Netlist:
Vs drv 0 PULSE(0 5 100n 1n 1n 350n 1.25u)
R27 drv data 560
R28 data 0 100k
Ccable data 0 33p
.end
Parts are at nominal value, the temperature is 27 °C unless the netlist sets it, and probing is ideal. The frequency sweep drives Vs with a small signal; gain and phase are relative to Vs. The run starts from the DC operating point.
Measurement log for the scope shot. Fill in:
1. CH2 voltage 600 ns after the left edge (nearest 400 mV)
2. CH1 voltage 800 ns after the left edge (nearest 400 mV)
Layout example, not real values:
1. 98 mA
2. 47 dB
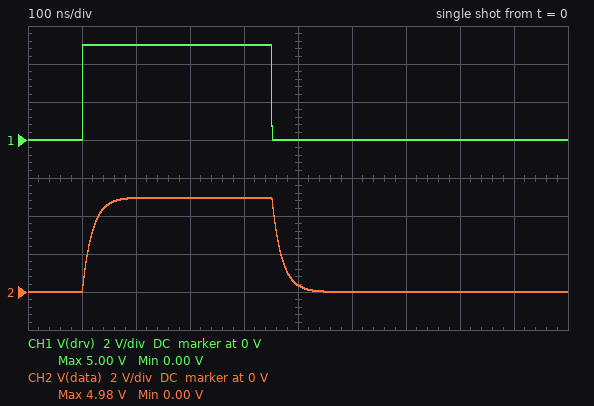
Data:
1. 0 V
2. 0 V
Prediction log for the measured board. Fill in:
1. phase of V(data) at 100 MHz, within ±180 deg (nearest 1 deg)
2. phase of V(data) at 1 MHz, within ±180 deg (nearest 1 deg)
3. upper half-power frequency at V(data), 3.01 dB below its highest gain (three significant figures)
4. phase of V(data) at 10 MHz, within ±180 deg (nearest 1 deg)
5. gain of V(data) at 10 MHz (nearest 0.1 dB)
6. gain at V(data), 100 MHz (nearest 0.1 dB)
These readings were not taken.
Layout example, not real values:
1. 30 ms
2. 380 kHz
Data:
1. -85 deg
2. -7 deg
3. 8.66 MHz
4. -49 deg
5. -3.7 dB
6. -21.3 dB
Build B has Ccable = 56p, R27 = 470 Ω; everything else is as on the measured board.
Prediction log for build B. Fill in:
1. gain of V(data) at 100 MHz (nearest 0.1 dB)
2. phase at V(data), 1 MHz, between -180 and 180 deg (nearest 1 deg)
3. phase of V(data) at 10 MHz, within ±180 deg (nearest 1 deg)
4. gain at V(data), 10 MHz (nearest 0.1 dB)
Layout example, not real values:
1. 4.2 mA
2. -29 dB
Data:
1. -24.4 dB
2. -9 deg
3. -59 deg
4. -5.7 dB
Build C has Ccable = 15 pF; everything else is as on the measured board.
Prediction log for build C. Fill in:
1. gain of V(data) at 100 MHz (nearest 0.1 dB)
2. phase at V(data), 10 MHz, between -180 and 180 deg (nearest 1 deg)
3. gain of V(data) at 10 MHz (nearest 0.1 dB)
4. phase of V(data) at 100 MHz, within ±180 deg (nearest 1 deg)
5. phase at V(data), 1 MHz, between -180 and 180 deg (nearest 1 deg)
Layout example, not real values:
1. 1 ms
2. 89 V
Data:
1. -14.6 dB
2. -28 deg
3. -1.1 dB
4. -79 deg
5. -3 deg
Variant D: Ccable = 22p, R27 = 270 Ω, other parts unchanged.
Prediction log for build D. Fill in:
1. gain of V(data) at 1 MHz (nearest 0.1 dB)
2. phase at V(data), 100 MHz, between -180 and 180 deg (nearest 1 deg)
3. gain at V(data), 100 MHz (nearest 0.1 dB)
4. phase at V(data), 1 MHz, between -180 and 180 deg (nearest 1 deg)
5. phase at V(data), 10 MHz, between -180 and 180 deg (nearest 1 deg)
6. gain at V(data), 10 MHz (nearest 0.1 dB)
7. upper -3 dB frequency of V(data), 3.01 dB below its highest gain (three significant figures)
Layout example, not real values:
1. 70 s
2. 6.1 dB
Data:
1. 0 dB
2. -75 deg
3. -11.7 dB
4. -2 deg
5. -20 deg
6. -0.6 dB
7. 26.9 MHz
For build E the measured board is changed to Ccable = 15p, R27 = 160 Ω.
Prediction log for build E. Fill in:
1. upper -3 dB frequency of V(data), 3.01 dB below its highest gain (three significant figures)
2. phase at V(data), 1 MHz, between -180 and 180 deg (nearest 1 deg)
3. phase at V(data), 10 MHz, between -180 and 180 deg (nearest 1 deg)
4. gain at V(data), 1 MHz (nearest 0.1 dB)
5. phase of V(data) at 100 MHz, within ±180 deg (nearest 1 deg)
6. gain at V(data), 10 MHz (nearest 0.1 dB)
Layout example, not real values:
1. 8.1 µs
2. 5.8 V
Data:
1. 66.4 MHz
2. -1 deg
3. -9 deg
4. 0 dB
5. -56 deg
6. -0.1 dB
